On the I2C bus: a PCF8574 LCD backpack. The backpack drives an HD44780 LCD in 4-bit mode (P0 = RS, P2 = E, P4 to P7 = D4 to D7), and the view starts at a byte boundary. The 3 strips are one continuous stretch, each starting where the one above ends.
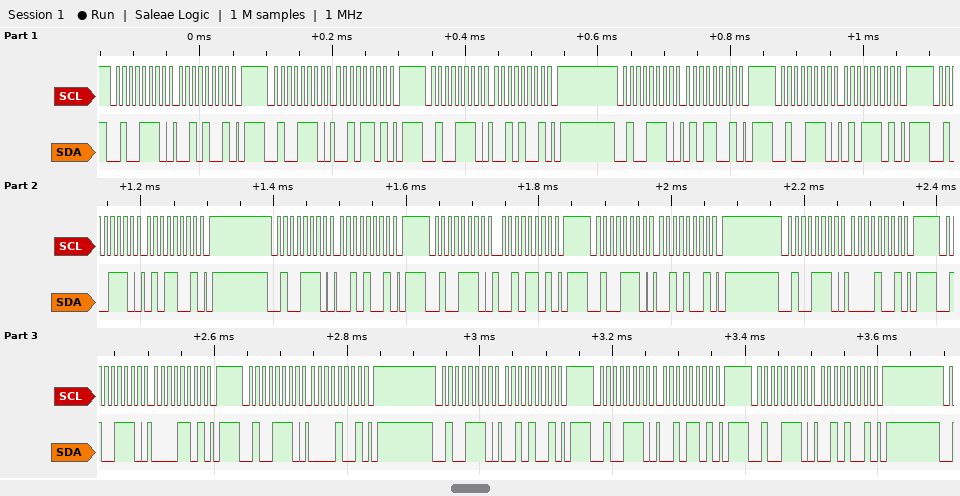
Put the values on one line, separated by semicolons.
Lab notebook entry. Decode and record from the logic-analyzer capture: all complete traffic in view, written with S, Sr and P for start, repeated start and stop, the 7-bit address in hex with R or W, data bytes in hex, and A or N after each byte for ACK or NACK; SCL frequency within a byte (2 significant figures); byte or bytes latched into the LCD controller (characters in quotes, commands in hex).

S 27W A 29 A P S 27W A 2D A P S 27W A 29 A P S 27W A 59 A P S 27W A 5D A P S 27W A 59 A P S 27W A 29 A P S 27W A 2D A P S 27W A 29 A P S 27W A 09 A P S 27W A 0D A P S 27W A 09 A P S 27W A 29 A P S 27W A 2D A P S 27W A 29 A P; 100 kHz; '%' ' '
